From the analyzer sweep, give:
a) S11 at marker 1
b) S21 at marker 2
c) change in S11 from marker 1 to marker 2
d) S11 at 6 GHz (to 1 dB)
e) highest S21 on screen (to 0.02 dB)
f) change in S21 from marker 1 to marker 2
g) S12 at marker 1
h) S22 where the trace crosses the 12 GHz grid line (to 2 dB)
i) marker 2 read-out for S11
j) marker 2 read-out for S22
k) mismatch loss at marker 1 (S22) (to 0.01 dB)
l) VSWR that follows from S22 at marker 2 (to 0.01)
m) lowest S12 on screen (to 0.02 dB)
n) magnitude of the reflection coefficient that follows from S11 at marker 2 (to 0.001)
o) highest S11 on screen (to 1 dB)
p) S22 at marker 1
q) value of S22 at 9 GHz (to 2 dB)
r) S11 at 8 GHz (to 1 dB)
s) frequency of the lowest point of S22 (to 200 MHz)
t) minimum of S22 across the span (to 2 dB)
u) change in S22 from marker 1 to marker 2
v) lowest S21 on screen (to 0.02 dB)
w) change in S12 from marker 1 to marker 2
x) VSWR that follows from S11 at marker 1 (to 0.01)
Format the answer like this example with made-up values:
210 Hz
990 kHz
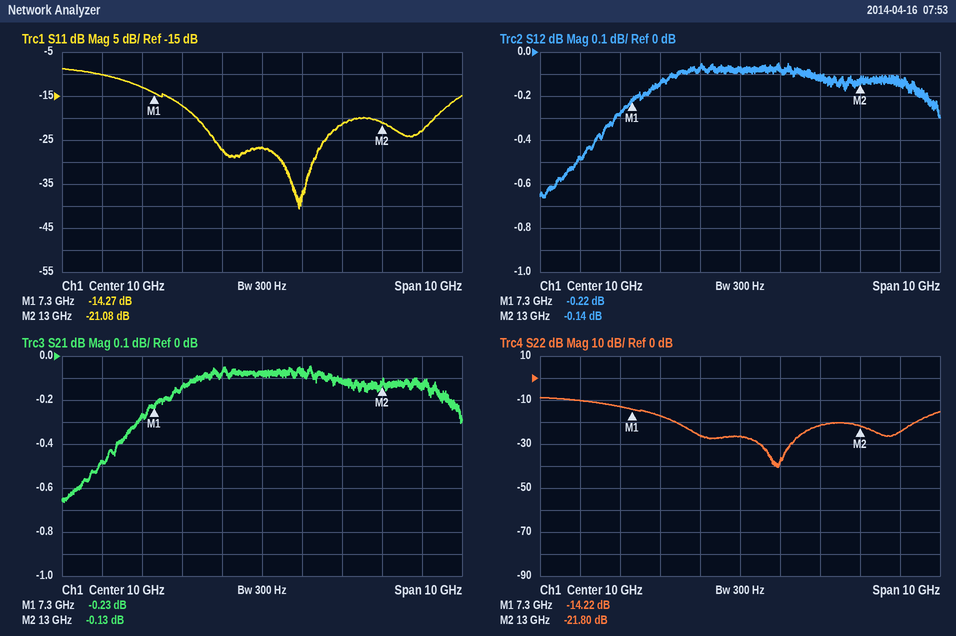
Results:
-14.27 dB
-0.13 dB
-6.81 dB
-10 dB
-0.04 dB
0.10 dB
-0.22 dB
-22 dB
-21.08 dB
-21.80 dB
0.17 dB
1.18
-0.66 dB
0.088
-9 dB
-14.22 dB
-26 dB
-17 dB
11.0 GHz
-40 dB
-7.58 dB
-0.66 dB
0.08 dB
1.48
